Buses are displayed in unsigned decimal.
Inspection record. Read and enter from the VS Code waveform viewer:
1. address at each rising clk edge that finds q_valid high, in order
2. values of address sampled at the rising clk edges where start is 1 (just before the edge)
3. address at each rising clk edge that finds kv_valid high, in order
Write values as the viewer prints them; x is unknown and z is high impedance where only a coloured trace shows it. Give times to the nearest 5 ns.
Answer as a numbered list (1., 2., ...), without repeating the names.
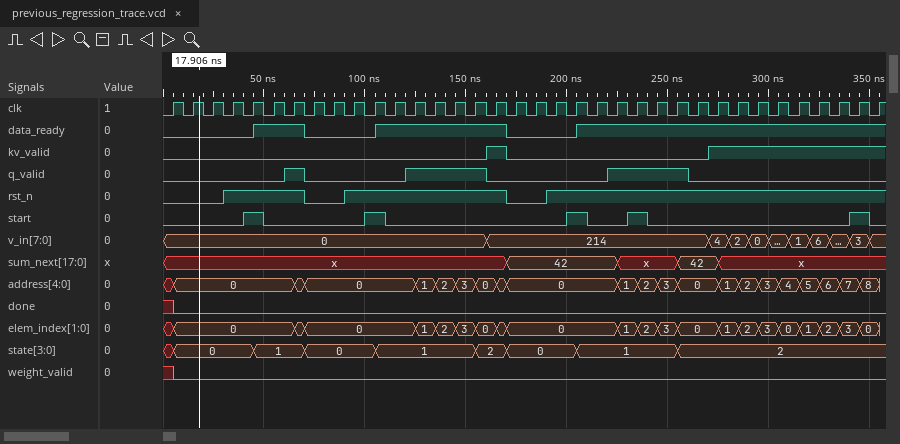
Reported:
1. 0, 0, 1, 2, 3, 0, 1, 2, 3
2. 0, 0, 0, 1, 7
3. 0, 0, 1, 2, 3, 4, 5, 6, 7, 8
